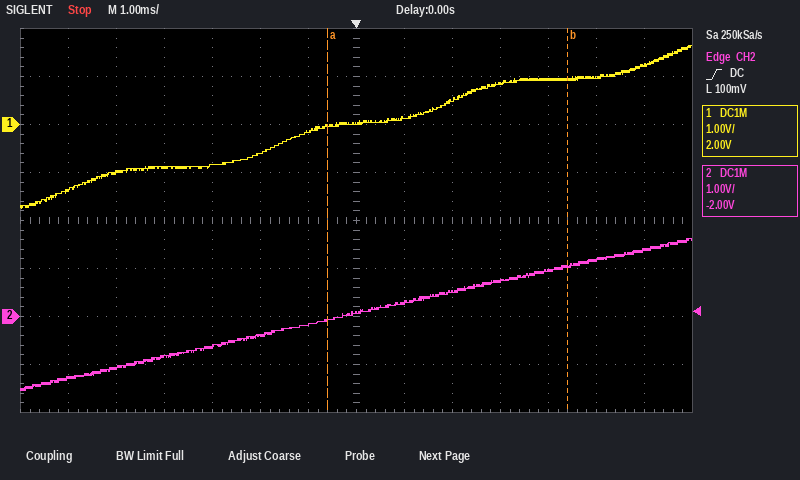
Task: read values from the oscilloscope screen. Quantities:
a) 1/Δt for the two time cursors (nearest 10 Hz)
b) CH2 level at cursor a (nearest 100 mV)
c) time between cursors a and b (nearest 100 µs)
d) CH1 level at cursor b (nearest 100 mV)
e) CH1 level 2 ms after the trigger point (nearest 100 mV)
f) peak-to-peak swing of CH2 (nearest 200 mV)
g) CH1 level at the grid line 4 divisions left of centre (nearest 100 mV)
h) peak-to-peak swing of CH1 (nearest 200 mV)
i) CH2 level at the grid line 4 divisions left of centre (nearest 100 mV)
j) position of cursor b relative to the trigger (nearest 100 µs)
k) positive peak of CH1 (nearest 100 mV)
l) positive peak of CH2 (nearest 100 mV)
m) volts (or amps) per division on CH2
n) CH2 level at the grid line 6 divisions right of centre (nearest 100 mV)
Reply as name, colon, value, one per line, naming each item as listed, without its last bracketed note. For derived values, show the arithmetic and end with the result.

1/Δt for the two time cursors: 1 / 5.0 ms ≈ 200 Hz
CH2 level at cursor a: -100 mV
time between cursors a and b: 5.0 ms
CH1 level at cursor b: 900 mV
CH1 level 2 ms after the trigger point: 500 mV
peak-to-peak swing of CH2: 3.2 V
CH1 level at the grid line 4 divisions left of centre: -900 mV
peak-to-peak swing of CH1: 3.4 V
CH2 level at the grid line 4 divisions left of centre: -800 mV
position of cursor b relative to the trigger: +4.4 ms
positive peak of CH1: 1.6 V
positive peak of CH2: 1.6 V
volts (or amps) per division on CH2: 1 V
CH2 level at the grid line 6 divisions right of centre: 1.4 V
